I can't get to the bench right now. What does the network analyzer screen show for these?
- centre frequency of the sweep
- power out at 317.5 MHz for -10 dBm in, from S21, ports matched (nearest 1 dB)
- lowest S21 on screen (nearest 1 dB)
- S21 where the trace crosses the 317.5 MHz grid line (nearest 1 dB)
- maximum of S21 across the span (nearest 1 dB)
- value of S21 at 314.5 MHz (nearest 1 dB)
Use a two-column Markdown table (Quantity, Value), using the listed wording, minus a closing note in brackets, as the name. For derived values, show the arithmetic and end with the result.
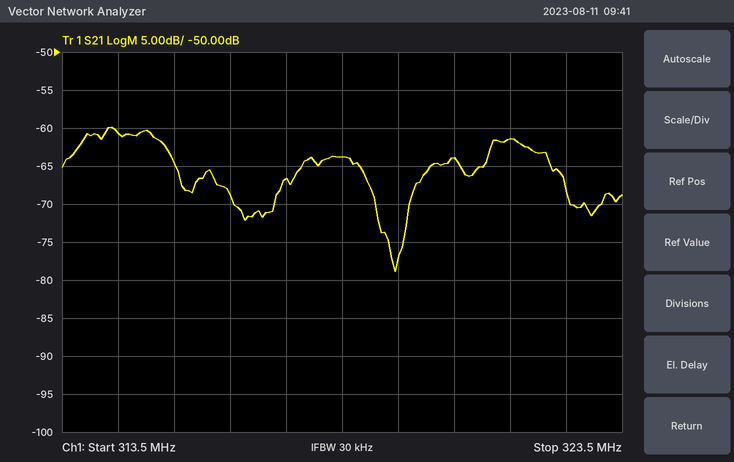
| Quantity | Value |
|---|---|
| centre frequency of the sweep | 318.5 MHz |
| power out at 317.5 MHz for -10 dBm in, from S21, ports matched | -10 dBm + (-67 dB) = -77 dBm |
| lowest S21 on screen | -79 dB |
| S21 where the trace crosses the 317.5 MHz grid line | -67 dB |
| maximum of S21 across the span | -60 dB |
| value of S21 at 314.5 MHz | -61 dB |
